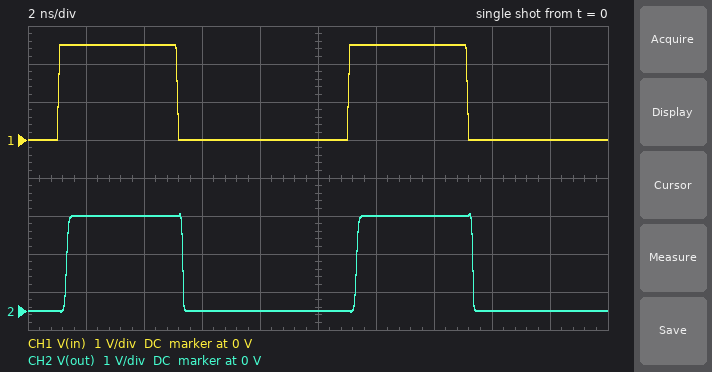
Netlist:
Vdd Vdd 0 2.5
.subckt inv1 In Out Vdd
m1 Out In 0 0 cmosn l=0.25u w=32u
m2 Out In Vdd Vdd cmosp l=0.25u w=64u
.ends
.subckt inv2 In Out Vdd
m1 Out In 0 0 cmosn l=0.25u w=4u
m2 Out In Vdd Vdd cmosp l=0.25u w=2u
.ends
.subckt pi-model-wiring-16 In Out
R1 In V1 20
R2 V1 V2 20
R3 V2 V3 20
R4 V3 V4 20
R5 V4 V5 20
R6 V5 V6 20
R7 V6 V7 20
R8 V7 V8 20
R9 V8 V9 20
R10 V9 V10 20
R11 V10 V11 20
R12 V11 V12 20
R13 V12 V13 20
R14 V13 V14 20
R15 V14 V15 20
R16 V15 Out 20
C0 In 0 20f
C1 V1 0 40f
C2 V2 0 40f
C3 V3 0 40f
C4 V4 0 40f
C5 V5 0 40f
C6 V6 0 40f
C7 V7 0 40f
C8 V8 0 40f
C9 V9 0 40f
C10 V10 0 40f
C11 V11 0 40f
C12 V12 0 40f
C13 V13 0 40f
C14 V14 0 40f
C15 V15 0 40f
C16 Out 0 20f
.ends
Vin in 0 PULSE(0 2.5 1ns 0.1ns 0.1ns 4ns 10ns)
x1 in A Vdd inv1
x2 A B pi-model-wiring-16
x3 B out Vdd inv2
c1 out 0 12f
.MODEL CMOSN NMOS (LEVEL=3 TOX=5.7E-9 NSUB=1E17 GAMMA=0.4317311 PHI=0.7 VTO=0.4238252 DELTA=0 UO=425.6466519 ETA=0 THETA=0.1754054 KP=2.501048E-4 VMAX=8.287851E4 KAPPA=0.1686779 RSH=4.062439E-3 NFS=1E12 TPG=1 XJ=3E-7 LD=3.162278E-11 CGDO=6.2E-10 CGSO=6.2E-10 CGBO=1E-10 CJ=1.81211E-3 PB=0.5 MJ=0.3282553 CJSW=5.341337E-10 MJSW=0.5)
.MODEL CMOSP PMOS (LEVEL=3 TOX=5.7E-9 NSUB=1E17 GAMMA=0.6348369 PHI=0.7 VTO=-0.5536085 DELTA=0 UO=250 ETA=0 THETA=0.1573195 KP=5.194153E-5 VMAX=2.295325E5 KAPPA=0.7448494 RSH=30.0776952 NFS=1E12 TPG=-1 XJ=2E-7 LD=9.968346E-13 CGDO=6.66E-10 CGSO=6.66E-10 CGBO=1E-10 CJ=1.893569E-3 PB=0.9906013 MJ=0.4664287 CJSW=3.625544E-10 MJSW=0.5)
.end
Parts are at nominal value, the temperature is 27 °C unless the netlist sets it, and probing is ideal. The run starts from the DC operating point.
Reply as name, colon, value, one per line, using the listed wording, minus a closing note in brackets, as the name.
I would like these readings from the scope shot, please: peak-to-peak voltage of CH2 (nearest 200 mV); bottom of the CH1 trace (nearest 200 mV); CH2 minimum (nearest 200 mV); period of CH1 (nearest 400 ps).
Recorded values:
peak-to-peak voltage of CH2: 2.6 V
bottom of the CH1 trace: 0 V
CH2 minimum: 0 V
period of CH1: 10.0 ns
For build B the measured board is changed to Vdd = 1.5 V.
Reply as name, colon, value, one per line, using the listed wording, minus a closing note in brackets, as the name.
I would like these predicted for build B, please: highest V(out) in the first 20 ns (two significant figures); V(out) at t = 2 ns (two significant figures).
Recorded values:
highest V(out) in the first 20 ns: 1.6 V
V(out) at t = 2 ns: 1.5 V
